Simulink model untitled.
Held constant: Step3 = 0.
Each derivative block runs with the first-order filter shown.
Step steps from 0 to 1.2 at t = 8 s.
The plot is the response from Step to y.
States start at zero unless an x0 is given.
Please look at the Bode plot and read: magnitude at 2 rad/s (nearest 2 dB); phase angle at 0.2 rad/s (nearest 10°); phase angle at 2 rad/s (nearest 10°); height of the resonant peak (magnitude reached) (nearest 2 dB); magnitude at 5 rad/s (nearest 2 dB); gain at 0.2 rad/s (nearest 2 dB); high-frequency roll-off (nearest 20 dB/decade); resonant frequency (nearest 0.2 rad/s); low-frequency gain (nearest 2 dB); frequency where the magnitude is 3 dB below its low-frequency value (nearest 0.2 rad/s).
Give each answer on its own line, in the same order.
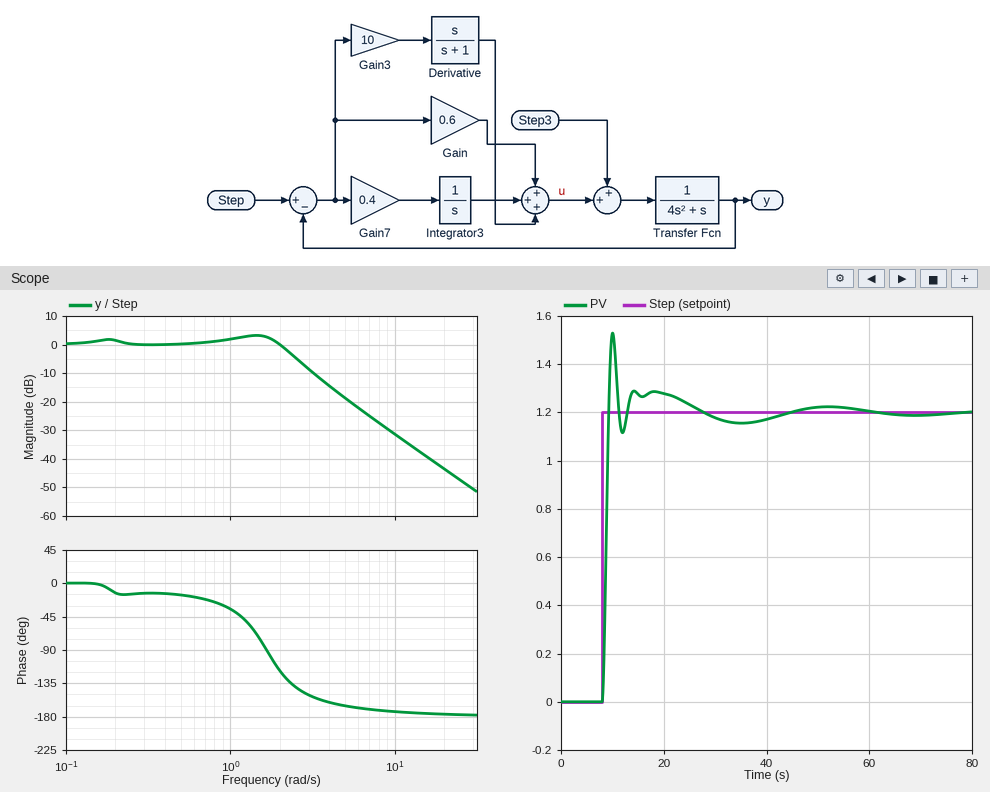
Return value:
0 dB
-10°
-120°
4 dB
-18 dB
2 dB
-40 dB/decade
1.4 rad/s
0 dB
2.2 rad/s
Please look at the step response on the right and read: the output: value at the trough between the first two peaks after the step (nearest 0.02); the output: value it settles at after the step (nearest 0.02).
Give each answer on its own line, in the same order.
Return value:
1.12
1.20
